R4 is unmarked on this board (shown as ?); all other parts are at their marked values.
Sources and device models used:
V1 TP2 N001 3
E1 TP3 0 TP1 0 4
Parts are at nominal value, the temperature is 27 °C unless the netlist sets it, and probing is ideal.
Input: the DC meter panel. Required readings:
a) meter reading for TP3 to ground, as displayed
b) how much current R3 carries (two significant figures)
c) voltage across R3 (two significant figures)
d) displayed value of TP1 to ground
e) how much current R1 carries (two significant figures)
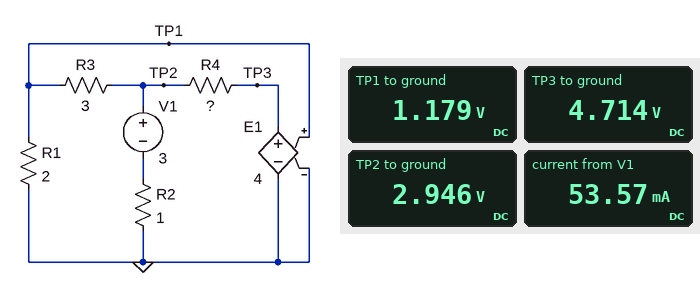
4.714 V
590 mA
1.8 V
1.179 V
590 mA
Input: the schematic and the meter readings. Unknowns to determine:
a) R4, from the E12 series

3.3 Ω
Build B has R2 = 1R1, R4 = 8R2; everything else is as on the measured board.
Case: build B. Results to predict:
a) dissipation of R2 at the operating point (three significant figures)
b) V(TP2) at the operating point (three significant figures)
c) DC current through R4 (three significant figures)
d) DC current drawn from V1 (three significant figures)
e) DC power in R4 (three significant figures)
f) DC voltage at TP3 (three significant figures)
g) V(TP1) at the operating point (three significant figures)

123 mW
2.63 V
193 mA
334 mA
304 mW
4.21 V
1.05 V
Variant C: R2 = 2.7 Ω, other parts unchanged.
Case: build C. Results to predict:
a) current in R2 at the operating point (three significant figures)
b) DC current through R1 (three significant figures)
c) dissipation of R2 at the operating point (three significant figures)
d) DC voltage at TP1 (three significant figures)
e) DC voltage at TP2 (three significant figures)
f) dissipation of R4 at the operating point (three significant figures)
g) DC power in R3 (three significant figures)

52.0 mA
572 mA
7.30 mW
1.14 V
2.86 V
892 mW
981 mW
